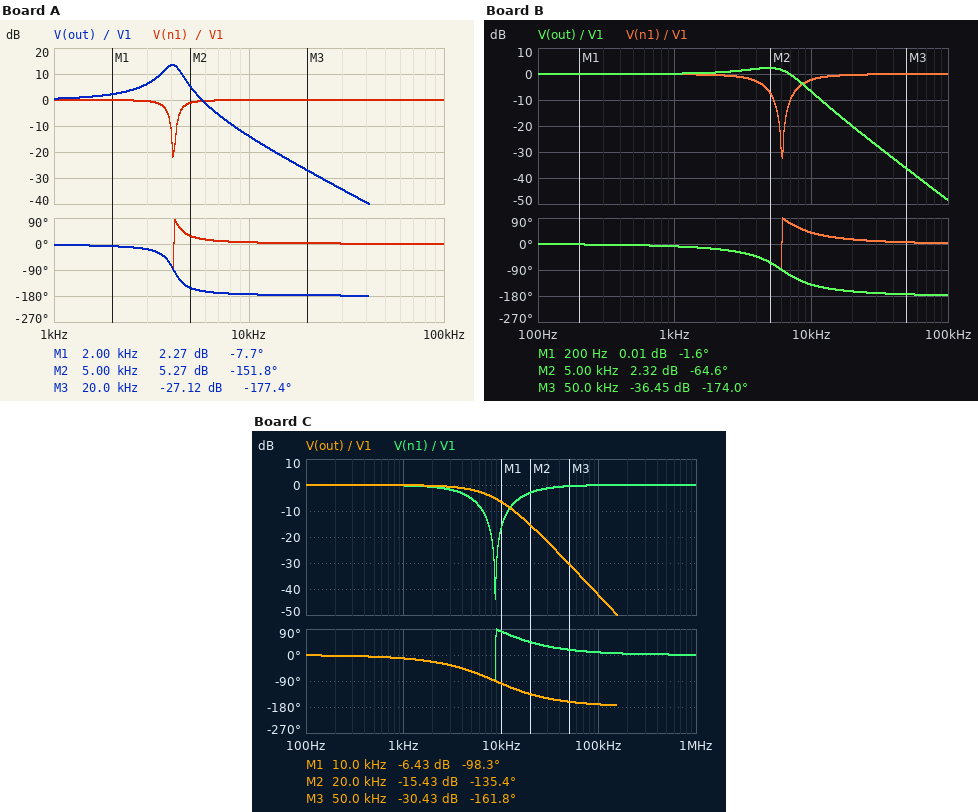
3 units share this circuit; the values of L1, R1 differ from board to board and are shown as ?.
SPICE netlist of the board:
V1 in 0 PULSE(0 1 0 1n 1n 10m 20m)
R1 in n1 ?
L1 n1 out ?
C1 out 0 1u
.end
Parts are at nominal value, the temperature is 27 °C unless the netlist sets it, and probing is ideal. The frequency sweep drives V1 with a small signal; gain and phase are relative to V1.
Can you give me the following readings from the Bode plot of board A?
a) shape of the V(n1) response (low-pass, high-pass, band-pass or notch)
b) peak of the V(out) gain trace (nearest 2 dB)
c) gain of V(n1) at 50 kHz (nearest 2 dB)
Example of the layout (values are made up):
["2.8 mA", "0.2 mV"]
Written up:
["notch", "14 dB", "0 dB"]
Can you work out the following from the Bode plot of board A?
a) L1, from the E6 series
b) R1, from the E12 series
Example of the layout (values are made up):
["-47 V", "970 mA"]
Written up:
["1.5 mH", "8.2 Ω"]
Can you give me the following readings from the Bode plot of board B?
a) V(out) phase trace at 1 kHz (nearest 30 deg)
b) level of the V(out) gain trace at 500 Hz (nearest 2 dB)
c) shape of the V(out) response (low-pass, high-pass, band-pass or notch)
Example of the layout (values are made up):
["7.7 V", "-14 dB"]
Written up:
["0 deg", "0 dB", "low-pass"]
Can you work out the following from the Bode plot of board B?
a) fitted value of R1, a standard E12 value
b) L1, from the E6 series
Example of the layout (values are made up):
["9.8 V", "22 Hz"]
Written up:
["22 Ω", "680 µH"]
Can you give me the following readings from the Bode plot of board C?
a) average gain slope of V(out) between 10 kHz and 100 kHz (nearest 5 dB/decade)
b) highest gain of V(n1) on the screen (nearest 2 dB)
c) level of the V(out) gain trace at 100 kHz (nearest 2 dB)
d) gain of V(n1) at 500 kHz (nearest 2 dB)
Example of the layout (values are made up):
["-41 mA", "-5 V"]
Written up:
["-35 dB/decade", "0 dB", "-42 dB", "0 dB"]
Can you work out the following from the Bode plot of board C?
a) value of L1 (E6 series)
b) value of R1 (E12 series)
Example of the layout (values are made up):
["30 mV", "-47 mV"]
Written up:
["330 µH", "33 Ω"]
